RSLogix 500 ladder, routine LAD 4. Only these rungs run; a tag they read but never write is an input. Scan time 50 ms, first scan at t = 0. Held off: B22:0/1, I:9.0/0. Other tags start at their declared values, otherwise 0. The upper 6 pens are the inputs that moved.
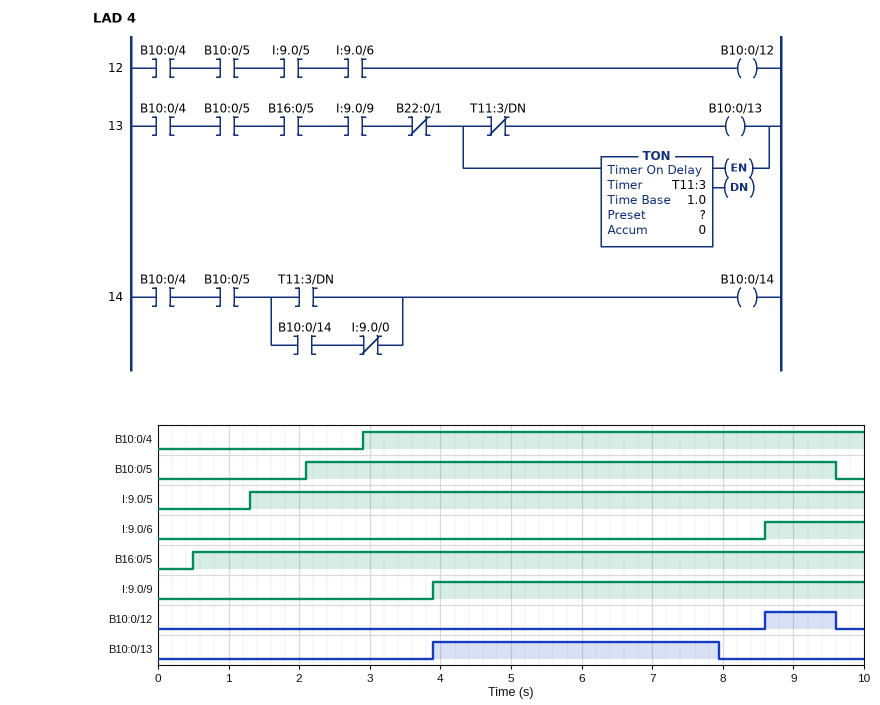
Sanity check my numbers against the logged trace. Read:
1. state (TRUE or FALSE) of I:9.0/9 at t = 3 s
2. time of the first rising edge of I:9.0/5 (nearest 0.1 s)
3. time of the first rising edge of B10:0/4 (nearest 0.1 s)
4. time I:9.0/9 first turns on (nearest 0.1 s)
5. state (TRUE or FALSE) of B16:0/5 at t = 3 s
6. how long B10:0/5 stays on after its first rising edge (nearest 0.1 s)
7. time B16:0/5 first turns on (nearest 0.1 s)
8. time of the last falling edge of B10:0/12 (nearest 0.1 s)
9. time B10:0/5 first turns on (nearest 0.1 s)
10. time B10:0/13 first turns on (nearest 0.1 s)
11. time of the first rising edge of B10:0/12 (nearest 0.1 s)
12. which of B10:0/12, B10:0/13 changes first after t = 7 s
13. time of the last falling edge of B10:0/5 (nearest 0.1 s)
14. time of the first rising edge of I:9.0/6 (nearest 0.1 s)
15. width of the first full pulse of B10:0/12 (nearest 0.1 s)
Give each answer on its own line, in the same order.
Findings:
FALSE
1.3 s
2.9 s
3.9 s
TRUE
7.5 s
0.5 s
9.6 s
2.1 s
3.9 s
8.6 s
B10:0/13
9.6 s
8.6 s
1.0 s
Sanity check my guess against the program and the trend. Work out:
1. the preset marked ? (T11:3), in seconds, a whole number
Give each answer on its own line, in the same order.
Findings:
4 s
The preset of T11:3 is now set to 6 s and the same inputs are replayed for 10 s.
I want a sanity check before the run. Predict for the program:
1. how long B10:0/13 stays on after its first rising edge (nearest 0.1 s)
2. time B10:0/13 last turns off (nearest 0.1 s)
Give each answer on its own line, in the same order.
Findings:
5.7 s
9.6 s
